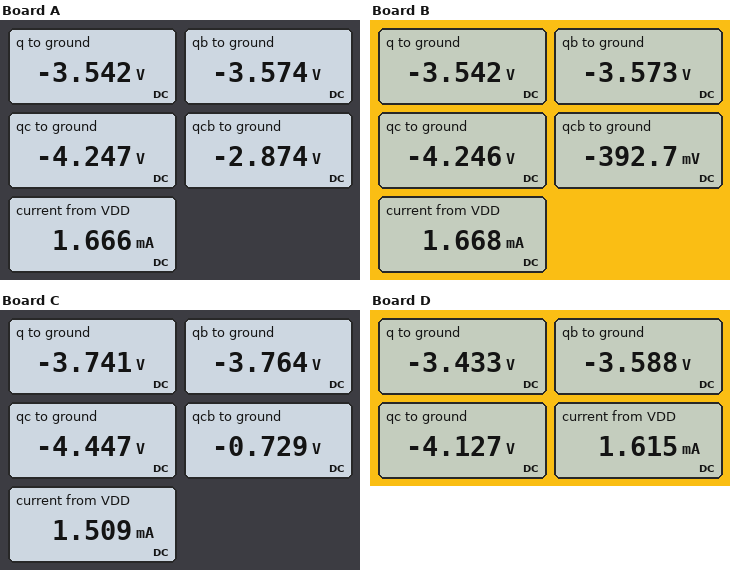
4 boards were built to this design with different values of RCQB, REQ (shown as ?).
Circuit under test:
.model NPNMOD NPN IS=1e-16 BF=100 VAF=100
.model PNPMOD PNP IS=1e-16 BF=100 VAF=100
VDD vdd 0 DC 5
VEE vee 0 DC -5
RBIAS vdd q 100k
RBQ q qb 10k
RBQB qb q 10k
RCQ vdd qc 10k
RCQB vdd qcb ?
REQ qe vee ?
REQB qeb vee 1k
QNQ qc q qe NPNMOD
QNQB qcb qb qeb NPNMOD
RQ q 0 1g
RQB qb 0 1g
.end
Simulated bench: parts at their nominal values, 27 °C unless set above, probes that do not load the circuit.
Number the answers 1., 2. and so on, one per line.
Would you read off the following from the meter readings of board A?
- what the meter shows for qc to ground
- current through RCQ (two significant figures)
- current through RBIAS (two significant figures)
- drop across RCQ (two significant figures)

1. -4.247 V
2. 920 µA
3. 85 µA
4. 9.2 V
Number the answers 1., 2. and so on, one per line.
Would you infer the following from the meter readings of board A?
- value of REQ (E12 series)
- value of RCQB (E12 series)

1. 680 Ω
2. 12 kΩ
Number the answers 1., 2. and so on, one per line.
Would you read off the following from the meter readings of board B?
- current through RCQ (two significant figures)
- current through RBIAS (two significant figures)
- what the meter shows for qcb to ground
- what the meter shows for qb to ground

1. 920 µA
2. 85 µA
3. -392.7 mV
4. -3.573 V
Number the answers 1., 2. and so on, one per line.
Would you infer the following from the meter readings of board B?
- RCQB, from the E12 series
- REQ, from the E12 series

1. 8.2 kΩ
2. 680 Ω
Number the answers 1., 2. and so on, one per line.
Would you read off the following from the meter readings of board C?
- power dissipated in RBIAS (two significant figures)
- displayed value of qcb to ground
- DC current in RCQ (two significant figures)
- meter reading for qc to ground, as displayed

1. 760 µW
2. -0.729 V
3. 940 µA
4. -4.447 V
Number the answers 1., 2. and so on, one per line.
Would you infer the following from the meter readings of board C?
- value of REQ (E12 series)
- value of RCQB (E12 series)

1. 470 Ω
2. 12 kΩ
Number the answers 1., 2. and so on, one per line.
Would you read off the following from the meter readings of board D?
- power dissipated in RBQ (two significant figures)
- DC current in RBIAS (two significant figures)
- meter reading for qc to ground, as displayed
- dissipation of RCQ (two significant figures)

1. 2.4 µW
2. 84 µA
3. -4.127 V
4. 8.3 mW
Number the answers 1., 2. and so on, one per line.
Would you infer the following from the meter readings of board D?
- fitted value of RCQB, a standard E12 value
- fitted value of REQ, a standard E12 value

1. 15 kΩ
2. 820 Ω
